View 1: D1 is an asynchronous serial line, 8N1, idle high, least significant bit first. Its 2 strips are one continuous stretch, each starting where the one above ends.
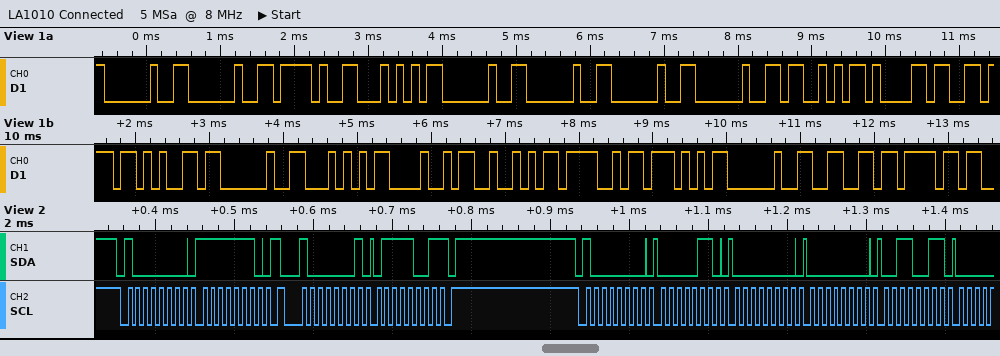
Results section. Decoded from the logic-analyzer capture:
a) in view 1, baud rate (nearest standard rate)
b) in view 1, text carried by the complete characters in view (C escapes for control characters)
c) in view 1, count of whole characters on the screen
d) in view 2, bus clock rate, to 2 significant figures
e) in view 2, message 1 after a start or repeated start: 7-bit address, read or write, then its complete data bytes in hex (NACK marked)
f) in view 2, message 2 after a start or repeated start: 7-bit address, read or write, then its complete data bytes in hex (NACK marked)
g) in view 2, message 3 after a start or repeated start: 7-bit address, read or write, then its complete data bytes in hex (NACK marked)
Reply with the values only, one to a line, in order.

9600 baud
"  /T    Save THROW fo"
21
100 kHz
0x40 write: FE
0x40 read: 79 NACK
0x40 write: 06 00 00 33
